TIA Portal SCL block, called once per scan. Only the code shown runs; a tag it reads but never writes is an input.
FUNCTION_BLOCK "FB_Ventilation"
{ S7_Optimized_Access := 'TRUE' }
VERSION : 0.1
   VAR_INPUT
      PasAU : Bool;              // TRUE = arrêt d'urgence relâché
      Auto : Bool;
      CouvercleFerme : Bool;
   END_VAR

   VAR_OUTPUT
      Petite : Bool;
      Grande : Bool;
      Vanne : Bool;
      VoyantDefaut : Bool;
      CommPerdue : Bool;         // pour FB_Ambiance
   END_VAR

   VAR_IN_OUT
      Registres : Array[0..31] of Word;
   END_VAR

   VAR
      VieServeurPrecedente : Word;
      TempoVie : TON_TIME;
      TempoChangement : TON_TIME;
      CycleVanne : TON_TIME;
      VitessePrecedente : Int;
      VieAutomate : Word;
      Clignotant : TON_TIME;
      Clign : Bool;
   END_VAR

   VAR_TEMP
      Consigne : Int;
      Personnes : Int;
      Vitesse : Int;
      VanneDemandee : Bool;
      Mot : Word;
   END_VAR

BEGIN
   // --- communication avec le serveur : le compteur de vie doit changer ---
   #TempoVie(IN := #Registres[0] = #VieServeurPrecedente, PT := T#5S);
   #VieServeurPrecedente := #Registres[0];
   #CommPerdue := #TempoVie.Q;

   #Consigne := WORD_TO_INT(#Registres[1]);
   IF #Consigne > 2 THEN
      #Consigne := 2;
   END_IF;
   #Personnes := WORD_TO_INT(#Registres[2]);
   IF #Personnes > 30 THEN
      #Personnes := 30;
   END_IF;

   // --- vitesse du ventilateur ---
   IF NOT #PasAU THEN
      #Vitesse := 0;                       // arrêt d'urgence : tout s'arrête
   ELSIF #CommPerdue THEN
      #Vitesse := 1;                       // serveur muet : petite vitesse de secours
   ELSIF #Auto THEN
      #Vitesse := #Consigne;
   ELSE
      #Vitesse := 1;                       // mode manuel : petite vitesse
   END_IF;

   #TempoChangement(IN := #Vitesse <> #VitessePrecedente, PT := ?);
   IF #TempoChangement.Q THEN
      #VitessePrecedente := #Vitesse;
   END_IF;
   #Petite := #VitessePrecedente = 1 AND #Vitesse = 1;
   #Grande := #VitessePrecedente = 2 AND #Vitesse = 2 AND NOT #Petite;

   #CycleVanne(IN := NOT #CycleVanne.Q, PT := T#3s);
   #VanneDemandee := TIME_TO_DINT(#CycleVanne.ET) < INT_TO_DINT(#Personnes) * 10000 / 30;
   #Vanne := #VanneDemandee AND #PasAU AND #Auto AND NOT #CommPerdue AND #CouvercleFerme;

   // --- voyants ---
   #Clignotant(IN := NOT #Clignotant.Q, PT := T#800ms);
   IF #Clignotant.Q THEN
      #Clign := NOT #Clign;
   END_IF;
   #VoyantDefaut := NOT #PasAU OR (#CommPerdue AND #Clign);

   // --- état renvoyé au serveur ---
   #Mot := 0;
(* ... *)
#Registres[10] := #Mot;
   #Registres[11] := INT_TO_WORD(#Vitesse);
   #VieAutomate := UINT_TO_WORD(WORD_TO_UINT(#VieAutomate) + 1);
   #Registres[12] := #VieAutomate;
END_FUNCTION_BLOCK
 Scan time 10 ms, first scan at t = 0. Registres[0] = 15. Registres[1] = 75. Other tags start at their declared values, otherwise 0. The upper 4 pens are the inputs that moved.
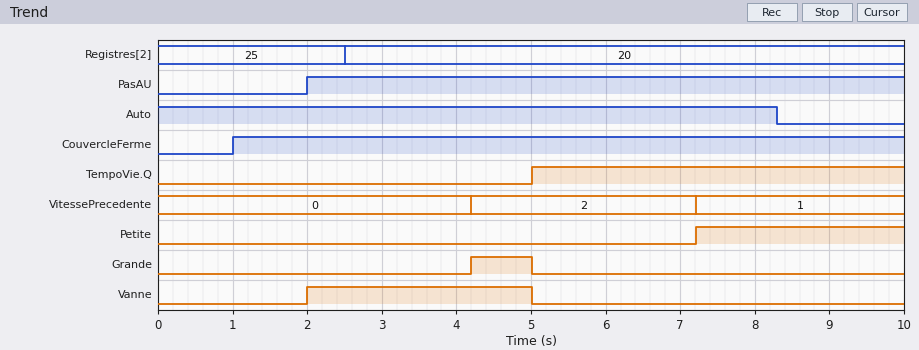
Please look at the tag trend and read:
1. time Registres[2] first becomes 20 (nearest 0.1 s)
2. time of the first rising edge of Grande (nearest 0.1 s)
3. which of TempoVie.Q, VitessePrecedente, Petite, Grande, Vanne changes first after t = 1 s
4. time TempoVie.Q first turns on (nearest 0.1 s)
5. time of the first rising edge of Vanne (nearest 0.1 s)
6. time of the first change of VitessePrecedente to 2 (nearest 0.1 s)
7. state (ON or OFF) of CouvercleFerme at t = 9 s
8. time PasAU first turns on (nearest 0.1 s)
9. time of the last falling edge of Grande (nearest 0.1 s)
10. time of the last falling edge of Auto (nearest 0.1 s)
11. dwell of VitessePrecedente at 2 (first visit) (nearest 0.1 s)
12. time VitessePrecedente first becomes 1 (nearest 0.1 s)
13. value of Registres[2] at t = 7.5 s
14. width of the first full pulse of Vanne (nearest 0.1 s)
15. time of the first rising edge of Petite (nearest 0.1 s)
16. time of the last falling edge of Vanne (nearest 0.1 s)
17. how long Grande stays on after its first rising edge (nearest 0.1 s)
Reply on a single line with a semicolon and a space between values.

2.5 s; 4.2 s; Vanne; 5.0 s; 2.0 s; 4.2 s; ON; 2.0 s; 5.0 s; 8.3 s; 3.0 s; 7.2 s; 20; 3.0 s; 7.2 s; 5.0 s; 0.8 s
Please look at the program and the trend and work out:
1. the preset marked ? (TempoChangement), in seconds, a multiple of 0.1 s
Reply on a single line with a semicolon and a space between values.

2.2 s
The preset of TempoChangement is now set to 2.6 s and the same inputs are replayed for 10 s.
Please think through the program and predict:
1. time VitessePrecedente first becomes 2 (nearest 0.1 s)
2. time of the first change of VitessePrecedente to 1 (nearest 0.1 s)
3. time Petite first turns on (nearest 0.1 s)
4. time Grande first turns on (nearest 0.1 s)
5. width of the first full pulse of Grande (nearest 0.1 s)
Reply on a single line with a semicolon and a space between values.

4.6 s; 7.6 s; 7.6 s; 4.6 s; 0.4 s
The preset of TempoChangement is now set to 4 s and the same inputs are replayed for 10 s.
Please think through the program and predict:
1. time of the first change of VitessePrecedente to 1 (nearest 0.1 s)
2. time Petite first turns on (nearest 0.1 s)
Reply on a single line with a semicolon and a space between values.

6.0 s; 6.0 s
